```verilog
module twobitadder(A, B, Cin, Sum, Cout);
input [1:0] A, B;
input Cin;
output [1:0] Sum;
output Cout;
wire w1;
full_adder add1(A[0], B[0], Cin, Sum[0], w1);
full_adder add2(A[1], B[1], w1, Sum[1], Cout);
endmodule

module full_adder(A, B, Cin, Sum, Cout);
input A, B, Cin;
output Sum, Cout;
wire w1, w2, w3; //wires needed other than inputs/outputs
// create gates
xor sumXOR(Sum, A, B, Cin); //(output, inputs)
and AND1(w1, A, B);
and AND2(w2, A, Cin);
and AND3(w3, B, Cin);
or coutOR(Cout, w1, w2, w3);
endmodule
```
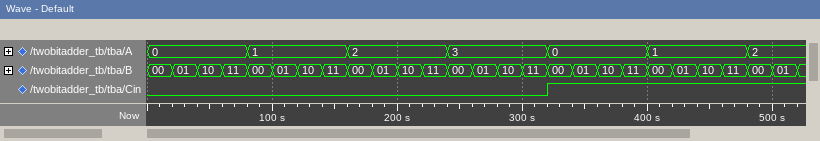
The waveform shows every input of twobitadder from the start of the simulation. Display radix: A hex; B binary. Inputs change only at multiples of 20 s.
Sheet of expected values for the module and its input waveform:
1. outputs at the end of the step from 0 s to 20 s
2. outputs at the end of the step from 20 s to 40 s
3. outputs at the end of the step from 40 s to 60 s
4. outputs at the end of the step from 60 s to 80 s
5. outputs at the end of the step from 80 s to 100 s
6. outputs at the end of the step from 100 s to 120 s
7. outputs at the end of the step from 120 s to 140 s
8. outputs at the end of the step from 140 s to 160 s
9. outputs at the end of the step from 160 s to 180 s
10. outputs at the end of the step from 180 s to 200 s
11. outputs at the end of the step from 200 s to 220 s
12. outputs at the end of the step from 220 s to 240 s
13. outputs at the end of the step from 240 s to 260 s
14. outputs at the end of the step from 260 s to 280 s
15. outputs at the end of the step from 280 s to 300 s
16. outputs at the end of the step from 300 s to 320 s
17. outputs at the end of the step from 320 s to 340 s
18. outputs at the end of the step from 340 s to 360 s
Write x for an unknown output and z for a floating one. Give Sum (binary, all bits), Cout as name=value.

Sum=00, Cout=0
Sum=01, Cout=0
Sum=10, Cout=0
Sum=11, Cout=0
Sum=01, Cout=0
Sum=10, Cout=0
Sum=11, Cout=0
Sum=00, Cout=1
Sum=10, Cout=0
Sum=11, Cout=0
Sum=00, Cout=1
Sum=01, Cout=1
Sum=11, Cout=0
Sum=00, Cout=1
Sum=01, Cout=1
Sum=10, Cout=1
Sum=01, Cout=0
Sum=10, Cout=0
